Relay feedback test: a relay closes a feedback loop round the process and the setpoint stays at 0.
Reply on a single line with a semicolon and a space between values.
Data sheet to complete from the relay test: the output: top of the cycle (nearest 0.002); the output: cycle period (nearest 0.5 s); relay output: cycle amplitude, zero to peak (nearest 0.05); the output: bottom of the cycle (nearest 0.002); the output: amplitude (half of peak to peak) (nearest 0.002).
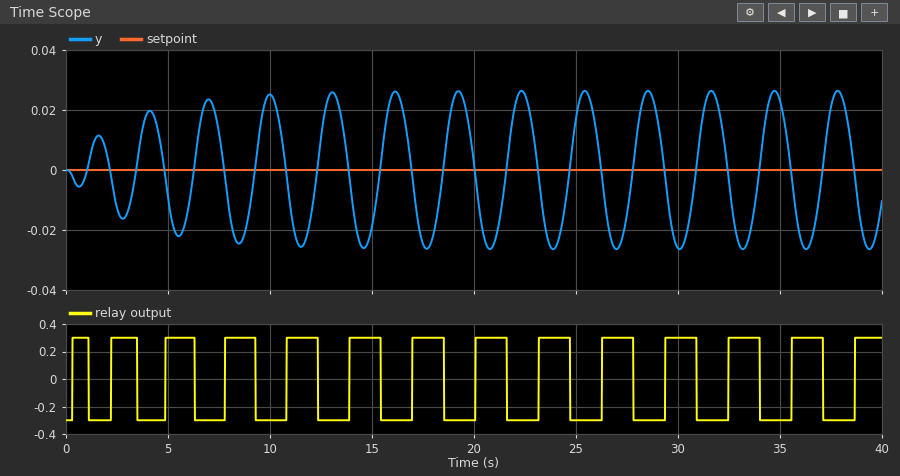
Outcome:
0.026; 3.0 s; 0.30; -0.026; 0.026
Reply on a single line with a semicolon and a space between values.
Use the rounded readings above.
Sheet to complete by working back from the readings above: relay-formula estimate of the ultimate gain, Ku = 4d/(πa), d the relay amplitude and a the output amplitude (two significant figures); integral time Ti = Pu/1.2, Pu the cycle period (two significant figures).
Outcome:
15; 2.5 s
